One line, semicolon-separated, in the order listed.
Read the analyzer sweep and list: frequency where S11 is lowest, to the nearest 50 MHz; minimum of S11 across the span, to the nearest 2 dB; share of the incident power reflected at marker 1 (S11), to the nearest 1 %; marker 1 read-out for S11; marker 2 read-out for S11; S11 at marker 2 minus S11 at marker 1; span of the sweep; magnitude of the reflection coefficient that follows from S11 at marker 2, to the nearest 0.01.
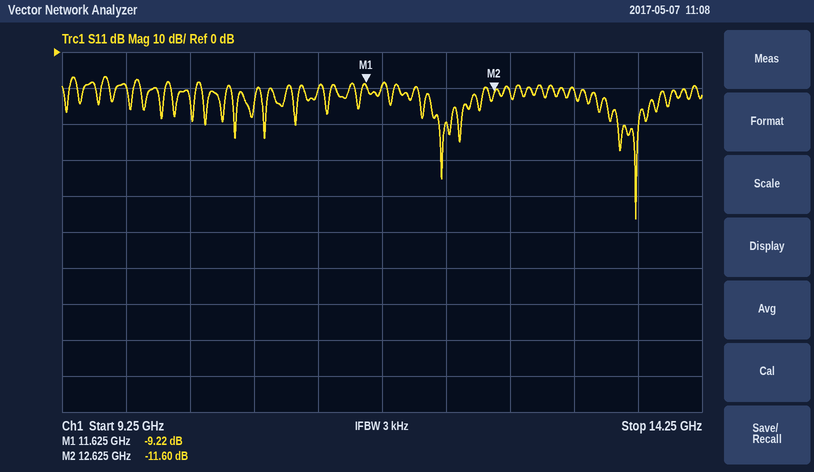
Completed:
13.75 GHz; -46 dB; 12 %; -9.22 dB; -11.60 dB; -2.38 dB; 5 GHz; 0.26
